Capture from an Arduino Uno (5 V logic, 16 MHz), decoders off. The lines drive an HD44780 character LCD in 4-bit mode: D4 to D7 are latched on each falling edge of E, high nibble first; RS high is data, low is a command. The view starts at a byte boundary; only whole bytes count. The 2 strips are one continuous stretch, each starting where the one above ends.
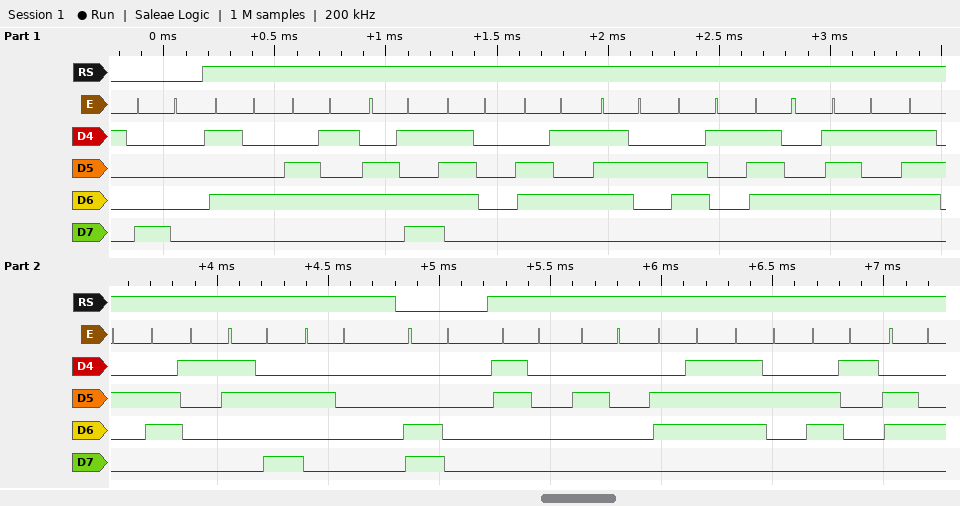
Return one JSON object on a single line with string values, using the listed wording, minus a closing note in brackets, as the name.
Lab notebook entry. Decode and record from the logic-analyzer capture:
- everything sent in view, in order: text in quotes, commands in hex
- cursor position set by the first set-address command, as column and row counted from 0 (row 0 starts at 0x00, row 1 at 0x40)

{"everything sent in view, in order: text in quotes, commands in hex": "0x80 \"Temperatura: \" 0xC0 \"0 grad\"", "cursor position set by the first set-address command, as column and row counted from 0": "column 0, row 0"}
